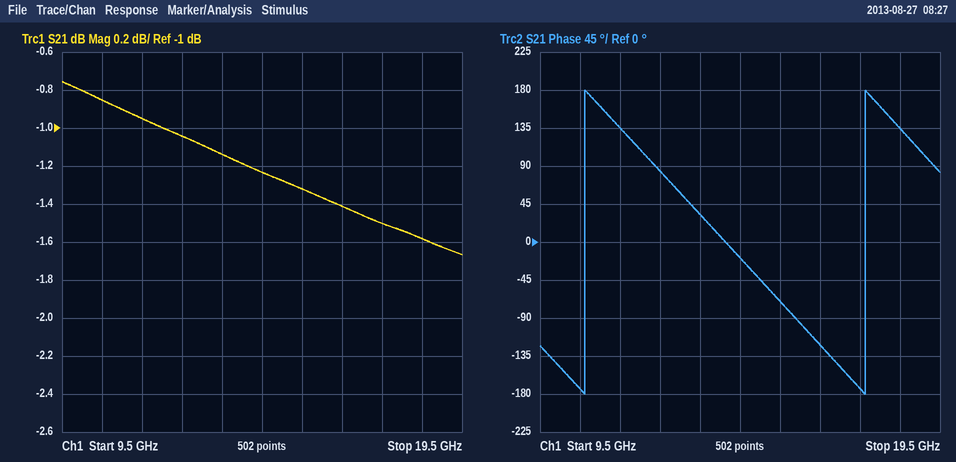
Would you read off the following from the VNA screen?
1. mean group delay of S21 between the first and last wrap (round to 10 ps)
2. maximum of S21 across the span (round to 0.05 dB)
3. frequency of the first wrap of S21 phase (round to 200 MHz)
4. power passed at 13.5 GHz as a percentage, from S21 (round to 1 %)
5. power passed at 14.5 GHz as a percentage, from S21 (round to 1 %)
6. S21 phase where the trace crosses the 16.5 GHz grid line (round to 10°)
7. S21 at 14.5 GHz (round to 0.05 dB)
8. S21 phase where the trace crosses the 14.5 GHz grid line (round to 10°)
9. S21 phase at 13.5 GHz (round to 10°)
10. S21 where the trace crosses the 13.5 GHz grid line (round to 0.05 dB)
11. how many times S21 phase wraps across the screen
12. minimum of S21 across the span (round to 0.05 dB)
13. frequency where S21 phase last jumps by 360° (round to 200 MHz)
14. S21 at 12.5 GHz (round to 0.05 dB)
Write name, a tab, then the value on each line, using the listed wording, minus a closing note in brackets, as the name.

mean group delay of S21 between the first and last wrap	140 ps
maximum of S21 across the span	-0.75 dB
frequency of the first wrap of S21 phase	10.6 GHz
power passed at 13.5 GHz as a percentage, from S21	77 %
power passed at 14.5 GHz as a percentage, from S21	75 %
S21 phase where the trace crosses the 16.5 GHz grid line	-120°
S21 at 14.5 GHz	-1.25 dB
S21 phase where the trace crosses the 14.5 GHz grid line	-20°
S21 phase at 13.5 GHz	30°
S21 where the trace crosses the 13.5 GHz grid line	-1.15 dB
how many times S21 phase wraps across the screen	2
minimum of S21 across the span	-1.65 dB
frequency where S21 phase last jumps by 360°	17.6 GHz
S21 at 12.5 GHz	-1.05 dB
